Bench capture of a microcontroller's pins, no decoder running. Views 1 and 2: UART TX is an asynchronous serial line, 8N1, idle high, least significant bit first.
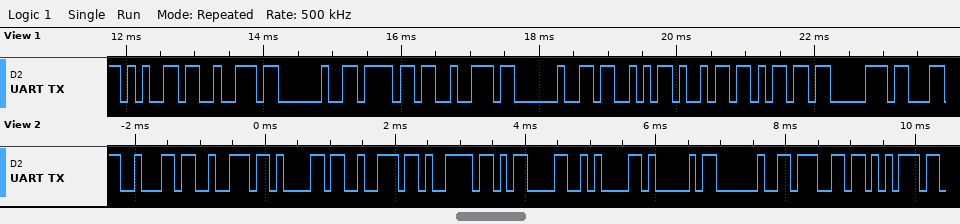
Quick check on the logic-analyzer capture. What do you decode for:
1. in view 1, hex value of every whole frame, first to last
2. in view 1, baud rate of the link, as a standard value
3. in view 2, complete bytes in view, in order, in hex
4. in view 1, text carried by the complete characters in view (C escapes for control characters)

0x65 0x72 0x20 0x6F 0x72 0x20 0x53 0x69 0x6D 0x70
9600 baud
62 72 61 72 79 0D 0A 41 20 67 75
"er or Simp"
